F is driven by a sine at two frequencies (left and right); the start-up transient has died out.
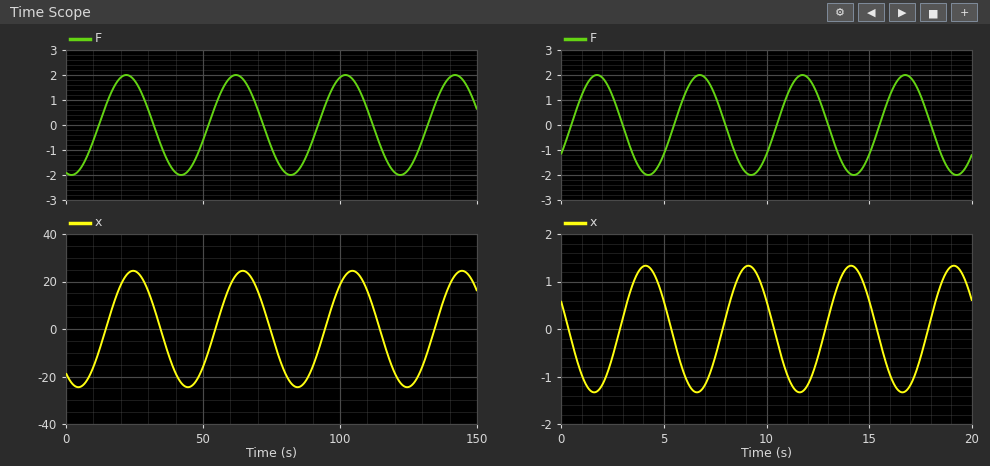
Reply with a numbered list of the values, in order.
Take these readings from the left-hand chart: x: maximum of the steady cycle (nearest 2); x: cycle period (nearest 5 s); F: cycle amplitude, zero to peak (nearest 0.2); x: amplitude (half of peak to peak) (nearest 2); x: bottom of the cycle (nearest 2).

1. 24
2. 40 s
3. 2.0
4. 24
5. -24
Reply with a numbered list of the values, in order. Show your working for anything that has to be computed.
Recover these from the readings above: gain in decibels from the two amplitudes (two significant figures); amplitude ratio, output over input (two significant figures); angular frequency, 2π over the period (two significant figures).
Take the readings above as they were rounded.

1. 20 log10(24 / 2) = 22 dB
2. 24 / 2 = 12
3. 2π / 40 = 0.16 rad/s
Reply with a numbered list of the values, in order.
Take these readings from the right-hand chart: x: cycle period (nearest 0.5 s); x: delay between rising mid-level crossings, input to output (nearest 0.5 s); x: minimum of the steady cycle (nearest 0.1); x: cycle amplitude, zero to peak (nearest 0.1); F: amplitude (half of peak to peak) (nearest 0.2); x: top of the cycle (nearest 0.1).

1. 5.0 s
2. 2.5 s
3. -1.3
4. 1.3
5. 2.0
6. 1.3
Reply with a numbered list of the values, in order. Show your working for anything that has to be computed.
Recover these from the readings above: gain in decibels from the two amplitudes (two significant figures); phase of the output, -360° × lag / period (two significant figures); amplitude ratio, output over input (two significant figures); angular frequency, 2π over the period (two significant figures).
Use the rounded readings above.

1. 20 log10(1.3 / 2) = -3.7 dB
2. -360 × 2.5 / 5 = -180°
3. 1.3 / 2 = 0.65
4. 2π / 5 = 1.3 rad/s
